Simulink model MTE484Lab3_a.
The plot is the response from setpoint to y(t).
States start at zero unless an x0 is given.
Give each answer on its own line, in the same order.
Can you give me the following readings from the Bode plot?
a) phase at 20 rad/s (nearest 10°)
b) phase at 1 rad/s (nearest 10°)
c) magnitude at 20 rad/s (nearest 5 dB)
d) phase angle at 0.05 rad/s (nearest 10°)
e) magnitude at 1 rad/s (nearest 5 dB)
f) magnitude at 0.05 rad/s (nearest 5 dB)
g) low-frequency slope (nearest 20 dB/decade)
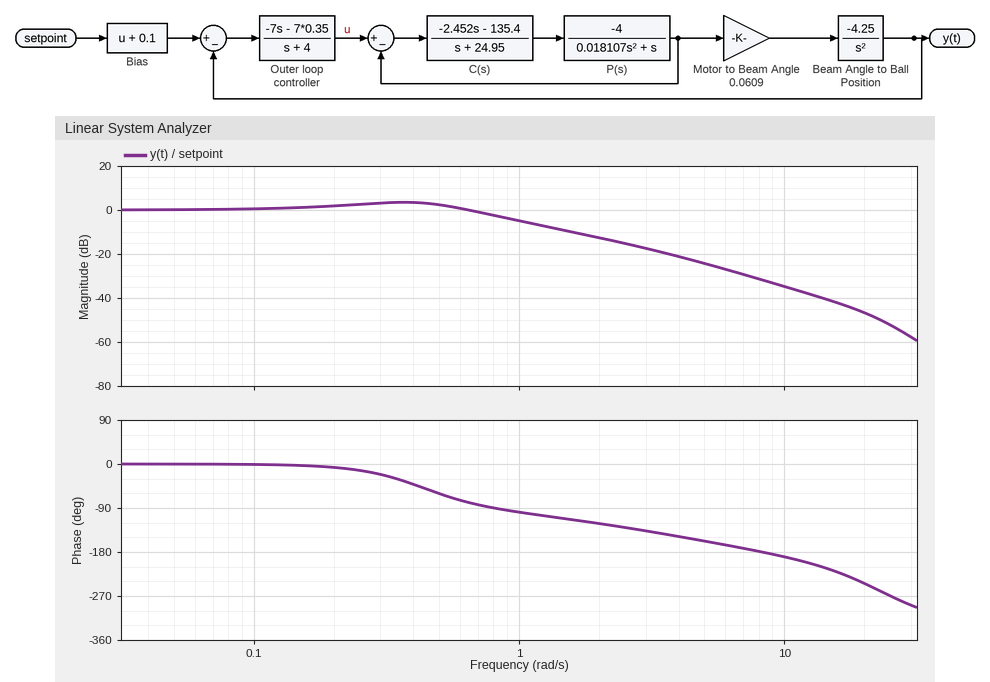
-240°
-100°
-45 dB
0°
-5 dB
0 dB
0 dB/decade
